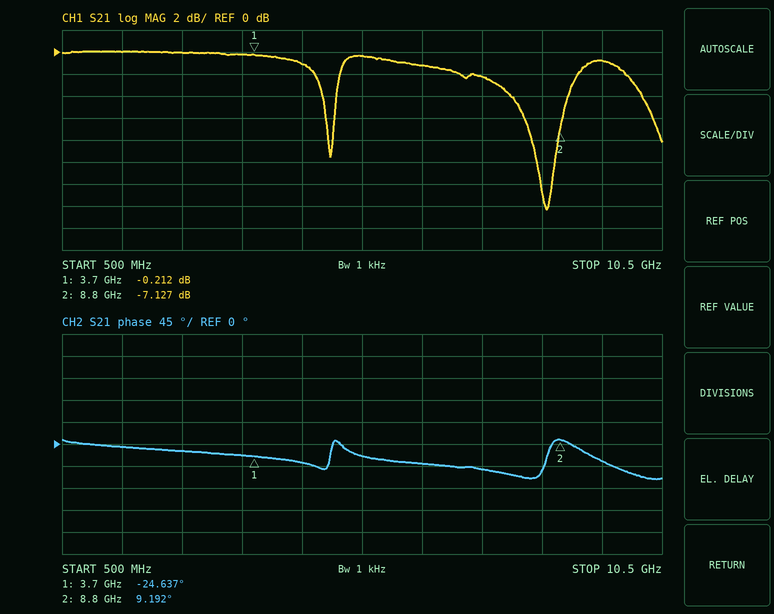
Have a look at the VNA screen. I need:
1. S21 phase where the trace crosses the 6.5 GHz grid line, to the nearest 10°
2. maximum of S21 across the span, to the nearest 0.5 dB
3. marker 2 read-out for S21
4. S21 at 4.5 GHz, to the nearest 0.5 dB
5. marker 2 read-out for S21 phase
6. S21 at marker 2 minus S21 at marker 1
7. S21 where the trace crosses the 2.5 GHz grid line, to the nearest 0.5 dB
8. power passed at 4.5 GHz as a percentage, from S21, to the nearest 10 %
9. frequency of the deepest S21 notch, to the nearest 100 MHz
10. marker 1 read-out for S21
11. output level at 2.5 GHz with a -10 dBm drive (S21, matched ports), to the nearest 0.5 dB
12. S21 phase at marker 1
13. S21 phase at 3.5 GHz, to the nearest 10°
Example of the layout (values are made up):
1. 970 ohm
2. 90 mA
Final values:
1. -40°
2. 0.0 dB
3. -7.127 dB
4. -1.0 dB
5. 9.192°
6. -6.915 dB
7. 0.0 dB
8. 80 %
9. 8.6 GHz
10. -0.212 dB
11. -10.0 dBm
12. -24.637°
13. -20°
